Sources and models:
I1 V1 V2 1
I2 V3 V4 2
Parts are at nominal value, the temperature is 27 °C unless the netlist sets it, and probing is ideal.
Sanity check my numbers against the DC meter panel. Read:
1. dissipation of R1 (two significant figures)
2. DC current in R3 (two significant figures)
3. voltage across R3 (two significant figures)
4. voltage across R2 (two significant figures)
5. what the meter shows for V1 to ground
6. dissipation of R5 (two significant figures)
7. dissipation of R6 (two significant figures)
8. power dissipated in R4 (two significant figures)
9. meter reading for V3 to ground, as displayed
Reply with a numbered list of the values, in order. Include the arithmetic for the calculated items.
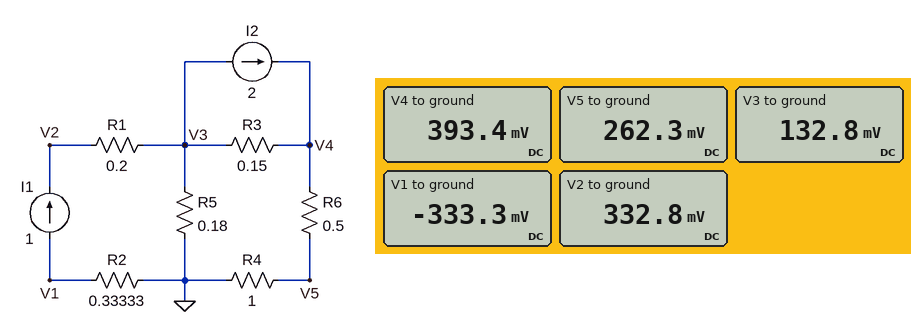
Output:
1. (332.8 mV - 132.8 mV)^2 / 200 mΩ = 200 mW
2. (393.4 mV - 132.8 mV) / 150 mΩ = 1.7 A
3. 393.4 mV - 132.8 mV = 260 mV
4. 0 V - (-333.3 mV) = 330 mV
5. -333.3 mV
6. (132.8 mV)^2 / 180 mΩ = 98 mW
7. (393.4 mV - 262.3 mV)^2 / 500 mΩ = 34 mW
8. (262.3 mV)^2 / 1 Ω = 69 mW
9. 132.8 mV
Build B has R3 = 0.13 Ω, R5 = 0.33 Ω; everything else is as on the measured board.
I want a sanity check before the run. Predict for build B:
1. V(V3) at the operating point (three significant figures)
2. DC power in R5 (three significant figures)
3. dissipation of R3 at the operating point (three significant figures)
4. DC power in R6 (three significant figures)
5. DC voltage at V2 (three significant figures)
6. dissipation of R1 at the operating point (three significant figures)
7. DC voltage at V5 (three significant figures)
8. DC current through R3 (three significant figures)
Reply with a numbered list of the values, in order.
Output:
1. 231 mV
2. 161 mW
3. 375 mW
4. 45.3 mW
5. 431 mV
6. 200 mW
7. 301 mV
8. 1.70 A
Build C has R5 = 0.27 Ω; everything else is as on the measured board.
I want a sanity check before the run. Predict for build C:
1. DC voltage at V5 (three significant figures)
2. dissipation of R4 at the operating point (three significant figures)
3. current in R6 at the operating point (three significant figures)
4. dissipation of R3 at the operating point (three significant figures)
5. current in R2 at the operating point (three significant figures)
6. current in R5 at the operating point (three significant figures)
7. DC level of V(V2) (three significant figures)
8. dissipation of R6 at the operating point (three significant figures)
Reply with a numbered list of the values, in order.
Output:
1. 297 mV
2. 88.1 mW
3. 297 mA
4. 435 mW
5. 1.00 A
6. 703 mA
7. 390 mV
8. 44.1 mW
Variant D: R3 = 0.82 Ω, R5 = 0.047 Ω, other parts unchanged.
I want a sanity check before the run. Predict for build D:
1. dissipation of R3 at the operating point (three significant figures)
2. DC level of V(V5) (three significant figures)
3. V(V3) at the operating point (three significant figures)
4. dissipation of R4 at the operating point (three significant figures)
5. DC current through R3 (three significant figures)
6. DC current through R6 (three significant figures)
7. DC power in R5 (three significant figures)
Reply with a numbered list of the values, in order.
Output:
1. 1.36 W
2. 713 mV
3. 13.5 mV
4. 508 mW
5. 1.29 A
6. 713 mA
7. 3.88 mW
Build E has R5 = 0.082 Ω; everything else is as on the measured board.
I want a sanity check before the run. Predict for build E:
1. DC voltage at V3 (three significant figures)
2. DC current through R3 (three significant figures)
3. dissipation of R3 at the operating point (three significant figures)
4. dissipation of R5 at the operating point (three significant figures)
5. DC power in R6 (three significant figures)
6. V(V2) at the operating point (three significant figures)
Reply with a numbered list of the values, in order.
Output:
1. 63.9 mV
2. 1.78 A
3. 475 mW
4. 49.8 mW
5. 24.3 mW
6. 264 mV
